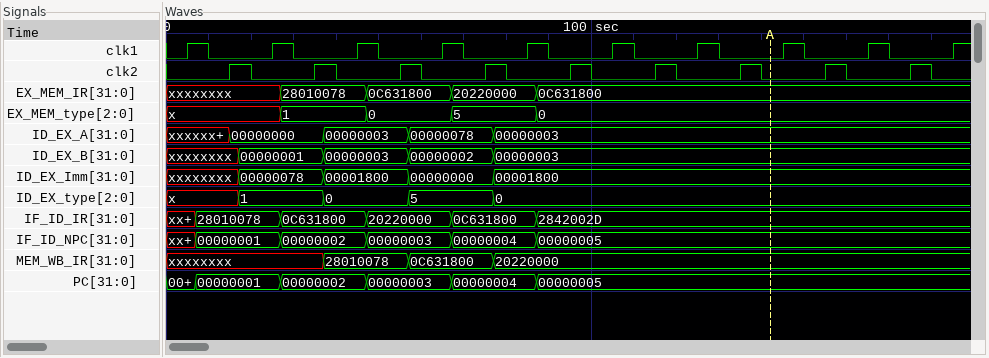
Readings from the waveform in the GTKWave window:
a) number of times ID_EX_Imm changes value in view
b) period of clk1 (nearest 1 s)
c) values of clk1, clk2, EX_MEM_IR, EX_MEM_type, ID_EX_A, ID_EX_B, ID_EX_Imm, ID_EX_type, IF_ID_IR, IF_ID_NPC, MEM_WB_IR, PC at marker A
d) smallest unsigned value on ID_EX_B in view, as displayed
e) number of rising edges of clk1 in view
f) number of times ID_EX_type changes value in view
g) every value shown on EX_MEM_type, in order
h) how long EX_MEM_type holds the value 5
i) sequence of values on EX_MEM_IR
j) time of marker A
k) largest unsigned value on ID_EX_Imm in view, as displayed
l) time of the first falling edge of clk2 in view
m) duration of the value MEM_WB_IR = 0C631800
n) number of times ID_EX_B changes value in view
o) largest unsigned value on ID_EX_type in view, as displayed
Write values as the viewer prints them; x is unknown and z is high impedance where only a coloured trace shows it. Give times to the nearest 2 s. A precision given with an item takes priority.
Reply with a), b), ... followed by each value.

a) 4
b) 20 s
c) clk1=0, clk2=0, EX_MEM_IR=0C631800, EX_MEM_type=0, ID_EX_A=00000003, ID_EX_B=00000003, ID_EX_Imm=00001800, ID_EX_type=0, IF_ID_IR=2842002D, IF_ID_NPC=00000005, MEM_WB_IR=20220000, PC=00000005
d) 00000001
e) 10
f) 4
g) x, 1, 0, 5, 0
h) 20 s
i) xxxxxxxx, 28010078, 0C631800, 20220000, 0C631800
j) 142 s
k) 00001800
l) 20 s
m) 20 s
n) 4
o) 5
